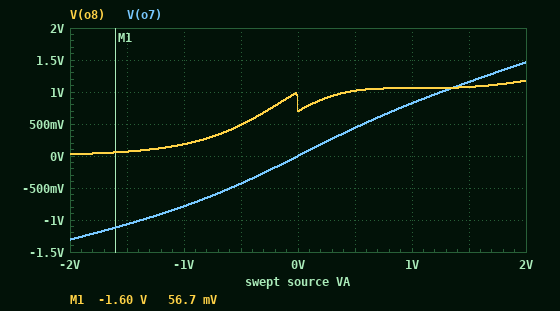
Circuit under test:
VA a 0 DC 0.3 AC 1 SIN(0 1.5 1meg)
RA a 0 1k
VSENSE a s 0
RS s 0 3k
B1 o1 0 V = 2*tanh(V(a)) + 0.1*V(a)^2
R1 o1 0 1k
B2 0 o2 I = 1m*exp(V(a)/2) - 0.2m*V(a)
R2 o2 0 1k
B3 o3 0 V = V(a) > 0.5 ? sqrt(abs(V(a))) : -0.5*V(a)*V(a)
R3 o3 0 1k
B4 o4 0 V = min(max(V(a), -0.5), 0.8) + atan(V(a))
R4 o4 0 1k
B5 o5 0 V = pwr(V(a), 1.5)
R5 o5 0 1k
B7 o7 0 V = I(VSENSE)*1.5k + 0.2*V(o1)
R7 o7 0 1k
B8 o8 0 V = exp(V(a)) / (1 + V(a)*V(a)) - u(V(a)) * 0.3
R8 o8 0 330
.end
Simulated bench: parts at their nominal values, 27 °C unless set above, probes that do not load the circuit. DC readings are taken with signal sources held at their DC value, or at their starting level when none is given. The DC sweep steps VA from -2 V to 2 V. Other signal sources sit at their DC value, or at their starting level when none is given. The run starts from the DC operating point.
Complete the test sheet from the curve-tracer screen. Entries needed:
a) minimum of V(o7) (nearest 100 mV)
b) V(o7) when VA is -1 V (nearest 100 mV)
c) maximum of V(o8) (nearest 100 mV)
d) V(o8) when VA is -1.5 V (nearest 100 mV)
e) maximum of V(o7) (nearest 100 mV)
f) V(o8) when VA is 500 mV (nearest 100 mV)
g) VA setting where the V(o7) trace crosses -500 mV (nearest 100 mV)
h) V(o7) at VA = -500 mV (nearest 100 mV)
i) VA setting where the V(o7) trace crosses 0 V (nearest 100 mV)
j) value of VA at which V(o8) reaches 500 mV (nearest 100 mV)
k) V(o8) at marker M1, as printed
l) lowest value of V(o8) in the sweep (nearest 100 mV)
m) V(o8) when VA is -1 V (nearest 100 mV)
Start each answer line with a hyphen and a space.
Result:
- -1.3 V
- -800 mV
- 1.2 V
- 100 mV
- 1.5 V
- 1.0 V
- -600 mV
- -400 mV
- 0 V
- -500 mV
- 56.7 mV
- 0 V
- 200 mV
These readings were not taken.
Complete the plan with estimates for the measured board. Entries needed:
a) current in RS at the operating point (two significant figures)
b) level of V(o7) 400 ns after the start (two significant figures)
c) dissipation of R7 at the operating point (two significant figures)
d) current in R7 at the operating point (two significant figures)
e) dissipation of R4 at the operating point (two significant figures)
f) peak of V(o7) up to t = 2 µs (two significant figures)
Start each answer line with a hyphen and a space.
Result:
- 100 µA
- 740 mV
- 72 µW
- 270 µA
- 350 µW
- 1.2 V
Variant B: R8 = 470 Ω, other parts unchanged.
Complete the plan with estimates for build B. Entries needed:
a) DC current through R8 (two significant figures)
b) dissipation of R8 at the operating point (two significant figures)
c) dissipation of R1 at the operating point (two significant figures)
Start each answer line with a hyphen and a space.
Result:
- 2.0 mA
- 1.9 mW
- 350 µW
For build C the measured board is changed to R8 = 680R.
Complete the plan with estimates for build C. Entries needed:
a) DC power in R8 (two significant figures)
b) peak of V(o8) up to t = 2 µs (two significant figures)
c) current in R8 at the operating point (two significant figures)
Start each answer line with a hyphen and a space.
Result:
- 1.3 mW
- 1.1 V
- 1.4 mA
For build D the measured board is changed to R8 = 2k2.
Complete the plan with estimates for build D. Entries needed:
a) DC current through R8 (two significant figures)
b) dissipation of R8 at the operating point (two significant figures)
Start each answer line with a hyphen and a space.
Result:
- 430 µA
- 400 µW
